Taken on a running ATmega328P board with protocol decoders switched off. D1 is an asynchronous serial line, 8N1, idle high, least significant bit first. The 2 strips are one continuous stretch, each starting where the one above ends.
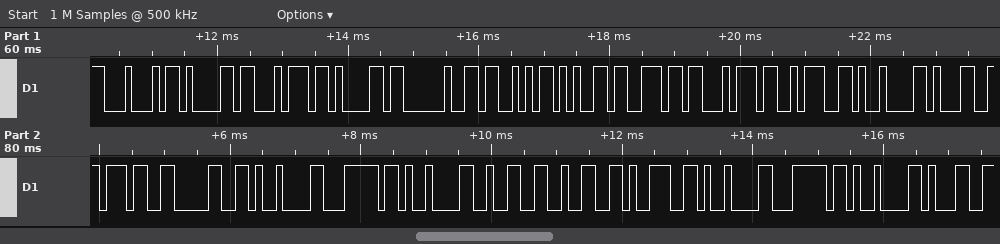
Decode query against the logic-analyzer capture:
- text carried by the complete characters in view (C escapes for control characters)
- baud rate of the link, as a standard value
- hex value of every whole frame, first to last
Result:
"Data Sent:\t170\t|\t229\t|\t1"
9600 baud
0x44 0x61 0x74 0x61 0x20 0x53 0x65 0x6E 0x74 0x3A 0x09 0x31 0x37 0x30 0x09 0x7C 0x09 0x32 0x32 0x39 0x09 0x7C 0x09 0x31
